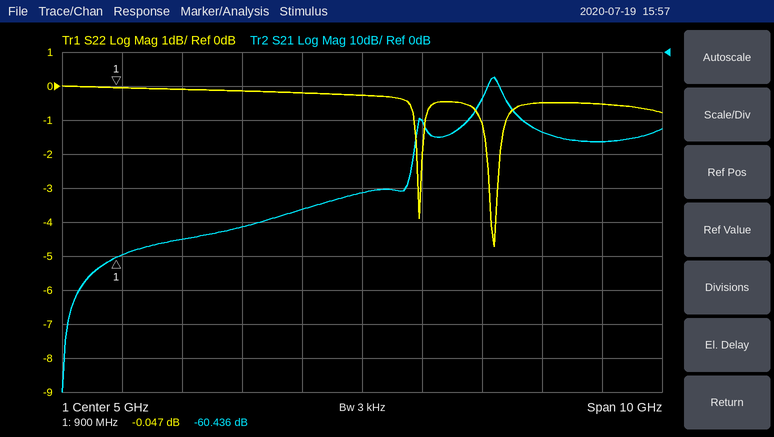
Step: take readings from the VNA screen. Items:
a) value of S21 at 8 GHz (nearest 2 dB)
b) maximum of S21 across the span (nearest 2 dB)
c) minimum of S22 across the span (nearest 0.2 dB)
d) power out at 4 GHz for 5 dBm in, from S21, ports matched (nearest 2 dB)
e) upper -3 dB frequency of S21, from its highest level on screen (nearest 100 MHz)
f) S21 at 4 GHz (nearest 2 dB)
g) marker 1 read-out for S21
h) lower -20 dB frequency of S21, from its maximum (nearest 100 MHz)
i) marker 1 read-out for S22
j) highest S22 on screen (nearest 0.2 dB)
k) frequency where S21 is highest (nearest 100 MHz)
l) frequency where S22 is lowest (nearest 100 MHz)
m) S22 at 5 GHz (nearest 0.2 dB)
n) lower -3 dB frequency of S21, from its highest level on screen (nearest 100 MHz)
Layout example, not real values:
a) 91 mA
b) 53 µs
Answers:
a) -24 dB
b) -8 dB
c) -4.8 dB
d) -42 dBm
e) 7.3 GHz
f) -46 dB
g) -60.436 dB
h) 5.9 GHz
i) -0.047 dB
j) 0.0 dB
k) 7.2 GHz
l) 7.2 GHz
m) -0.2 dB
n) 7.1 GHz
